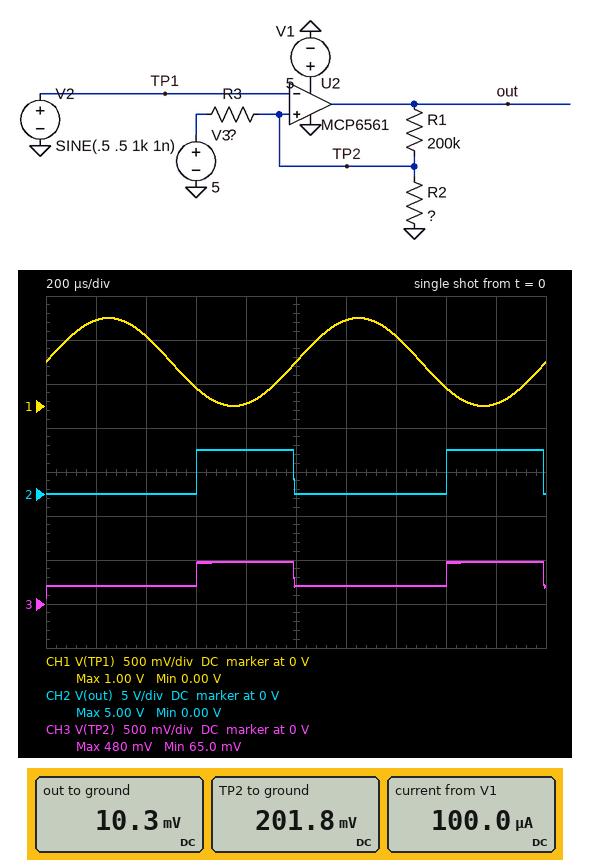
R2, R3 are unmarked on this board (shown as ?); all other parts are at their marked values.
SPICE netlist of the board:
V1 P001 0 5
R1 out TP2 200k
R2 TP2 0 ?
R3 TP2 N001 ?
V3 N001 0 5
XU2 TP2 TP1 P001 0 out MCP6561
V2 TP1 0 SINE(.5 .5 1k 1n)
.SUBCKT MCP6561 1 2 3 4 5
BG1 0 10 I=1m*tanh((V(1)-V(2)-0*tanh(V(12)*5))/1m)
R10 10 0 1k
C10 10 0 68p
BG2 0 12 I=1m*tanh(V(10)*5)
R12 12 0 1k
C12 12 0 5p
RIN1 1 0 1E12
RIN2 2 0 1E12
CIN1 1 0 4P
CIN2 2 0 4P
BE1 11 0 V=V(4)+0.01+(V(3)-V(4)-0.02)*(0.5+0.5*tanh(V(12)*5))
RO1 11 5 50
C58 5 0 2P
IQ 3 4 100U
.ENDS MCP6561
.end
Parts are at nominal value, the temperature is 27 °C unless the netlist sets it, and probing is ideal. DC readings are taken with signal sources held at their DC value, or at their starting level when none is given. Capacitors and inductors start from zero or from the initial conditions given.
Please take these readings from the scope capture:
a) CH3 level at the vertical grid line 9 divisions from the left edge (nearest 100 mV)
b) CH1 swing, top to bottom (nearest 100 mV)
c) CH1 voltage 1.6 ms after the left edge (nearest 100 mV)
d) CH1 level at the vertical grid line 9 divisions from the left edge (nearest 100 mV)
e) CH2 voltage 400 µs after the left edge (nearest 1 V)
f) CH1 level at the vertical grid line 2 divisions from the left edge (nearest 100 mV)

500 mV
1.0 V
200 mV
0 V
0 V
800 mV
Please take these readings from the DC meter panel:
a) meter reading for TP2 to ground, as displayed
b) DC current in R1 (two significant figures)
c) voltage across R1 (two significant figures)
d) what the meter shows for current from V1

201.8 mV
960 nA
190 mV
100.0 µA
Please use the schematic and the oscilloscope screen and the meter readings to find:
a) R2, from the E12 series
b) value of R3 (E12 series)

12 kΩ
270 kΩ
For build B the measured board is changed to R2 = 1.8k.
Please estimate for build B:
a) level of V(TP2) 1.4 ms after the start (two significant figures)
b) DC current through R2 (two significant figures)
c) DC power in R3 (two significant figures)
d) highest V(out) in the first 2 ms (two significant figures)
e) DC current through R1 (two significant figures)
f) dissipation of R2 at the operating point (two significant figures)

33 mV
18 µA
91 µW
5.0 V
110 nA
600 nW
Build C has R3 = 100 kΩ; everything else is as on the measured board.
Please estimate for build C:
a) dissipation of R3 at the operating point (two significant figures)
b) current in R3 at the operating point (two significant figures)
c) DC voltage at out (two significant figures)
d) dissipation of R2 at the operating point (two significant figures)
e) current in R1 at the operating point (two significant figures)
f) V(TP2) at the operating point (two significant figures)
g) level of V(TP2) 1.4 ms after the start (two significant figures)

180 µW
42 µA
5.0 V
48 µW
21 µA
760 mV
510 mV
